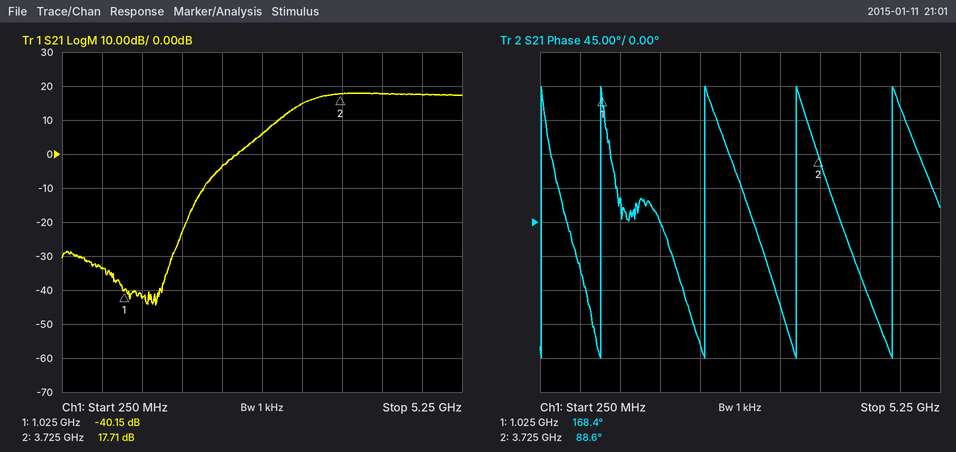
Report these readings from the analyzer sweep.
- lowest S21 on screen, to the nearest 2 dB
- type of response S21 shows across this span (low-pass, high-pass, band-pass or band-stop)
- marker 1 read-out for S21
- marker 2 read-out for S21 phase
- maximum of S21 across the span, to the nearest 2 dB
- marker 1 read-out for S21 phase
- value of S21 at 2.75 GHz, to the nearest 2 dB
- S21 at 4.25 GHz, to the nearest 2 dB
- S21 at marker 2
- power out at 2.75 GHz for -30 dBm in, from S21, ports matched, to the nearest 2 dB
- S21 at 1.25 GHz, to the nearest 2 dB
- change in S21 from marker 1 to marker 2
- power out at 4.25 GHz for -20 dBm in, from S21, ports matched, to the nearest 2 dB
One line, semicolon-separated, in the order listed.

-44 dB; high-pass; -40.15 dB; 88.6°; 18 dB; 168.4°; 6 dB; 18 dB; 17.71 dB; -24 dBm; -42 dB; 57.86 dB; -2 dBm
